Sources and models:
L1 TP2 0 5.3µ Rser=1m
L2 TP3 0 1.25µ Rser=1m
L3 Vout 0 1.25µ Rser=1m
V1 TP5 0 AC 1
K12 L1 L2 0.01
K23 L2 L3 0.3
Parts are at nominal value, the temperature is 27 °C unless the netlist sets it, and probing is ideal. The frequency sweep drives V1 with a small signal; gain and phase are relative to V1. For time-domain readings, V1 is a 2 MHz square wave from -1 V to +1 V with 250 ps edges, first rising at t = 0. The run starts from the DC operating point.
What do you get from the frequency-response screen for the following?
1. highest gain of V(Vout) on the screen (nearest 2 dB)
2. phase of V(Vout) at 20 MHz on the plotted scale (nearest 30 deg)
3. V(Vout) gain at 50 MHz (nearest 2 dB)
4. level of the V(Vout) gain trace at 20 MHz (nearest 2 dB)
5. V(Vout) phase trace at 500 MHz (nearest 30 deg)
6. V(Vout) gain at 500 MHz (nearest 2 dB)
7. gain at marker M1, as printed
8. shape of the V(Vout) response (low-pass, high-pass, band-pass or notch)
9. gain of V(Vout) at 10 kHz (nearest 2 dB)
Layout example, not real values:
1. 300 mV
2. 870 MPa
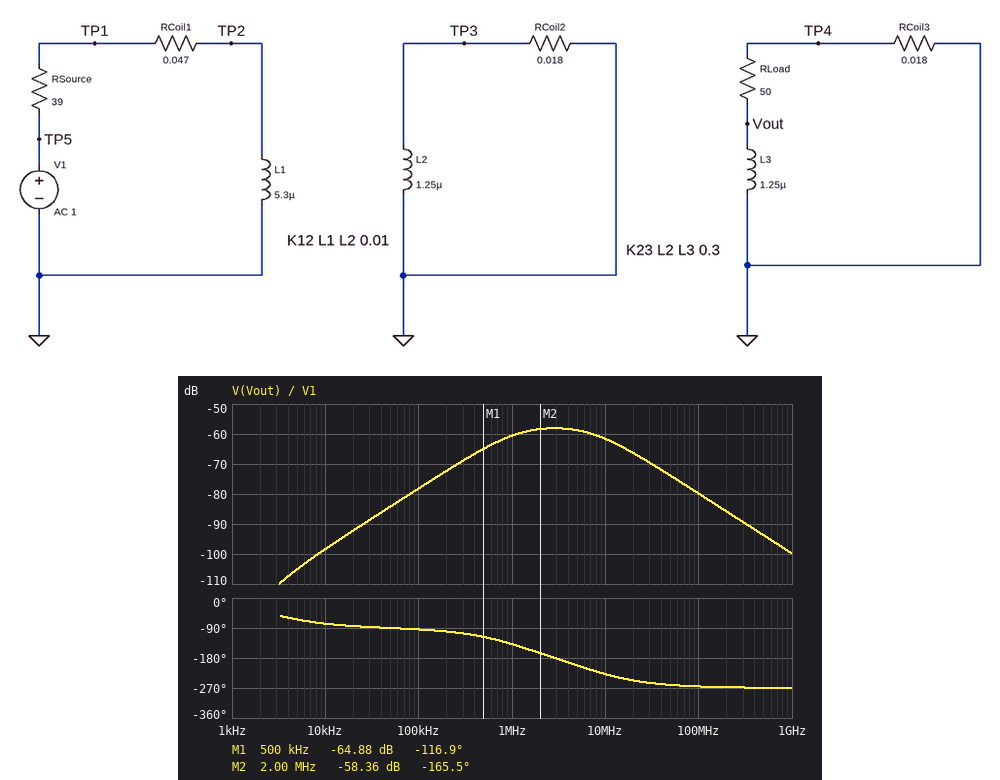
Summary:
1. -58 dB
2. -240 deg
3. -74 dB
4. -66 dB
5. -270 deg
6. -94 dB
7. -64.88 dB
8. band-pass
9. -98 dB
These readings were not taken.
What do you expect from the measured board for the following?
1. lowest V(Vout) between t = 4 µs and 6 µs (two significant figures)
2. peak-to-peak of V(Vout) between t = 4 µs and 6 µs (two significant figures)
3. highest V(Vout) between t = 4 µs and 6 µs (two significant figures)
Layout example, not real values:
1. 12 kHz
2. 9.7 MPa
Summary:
1. -1.7 mV
2. 3.4 mV
3. 1.7 mV
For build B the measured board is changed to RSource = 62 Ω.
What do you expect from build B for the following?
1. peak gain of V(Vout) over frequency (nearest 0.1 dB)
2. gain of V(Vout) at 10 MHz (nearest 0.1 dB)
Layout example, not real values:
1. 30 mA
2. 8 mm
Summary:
1. -58.8 dB
2. -61.7 dB
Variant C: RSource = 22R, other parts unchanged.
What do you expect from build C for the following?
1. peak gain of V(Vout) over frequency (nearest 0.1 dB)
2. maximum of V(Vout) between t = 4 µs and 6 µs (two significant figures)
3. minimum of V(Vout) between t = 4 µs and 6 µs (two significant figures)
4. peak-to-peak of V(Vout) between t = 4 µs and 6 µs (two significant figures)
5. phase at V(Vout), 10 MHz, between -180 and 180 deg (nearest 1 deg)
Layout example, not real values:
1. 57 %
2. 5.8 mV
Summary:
1. -57.5 dB
2. 1.6 mV
3. -1.6 mV
4. 3.3 mV
5. 129 deg
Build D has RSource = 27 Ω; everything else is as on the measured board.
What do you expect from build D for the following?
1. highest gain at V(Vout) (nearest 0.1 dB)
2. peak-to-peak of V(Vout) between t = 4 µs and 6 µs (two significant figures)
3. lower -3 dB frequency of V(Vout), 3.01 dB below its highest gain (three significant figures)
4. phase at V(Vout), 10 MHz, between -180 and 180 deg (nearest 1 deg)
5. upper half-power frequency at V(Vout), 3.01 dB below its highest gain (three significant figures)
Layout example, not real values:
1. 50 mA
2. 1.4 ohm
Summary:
1. -57.7 dB
2. 3.3 mV
3. 670 kHz
4. 130 deg
5. 8.48 MHz
